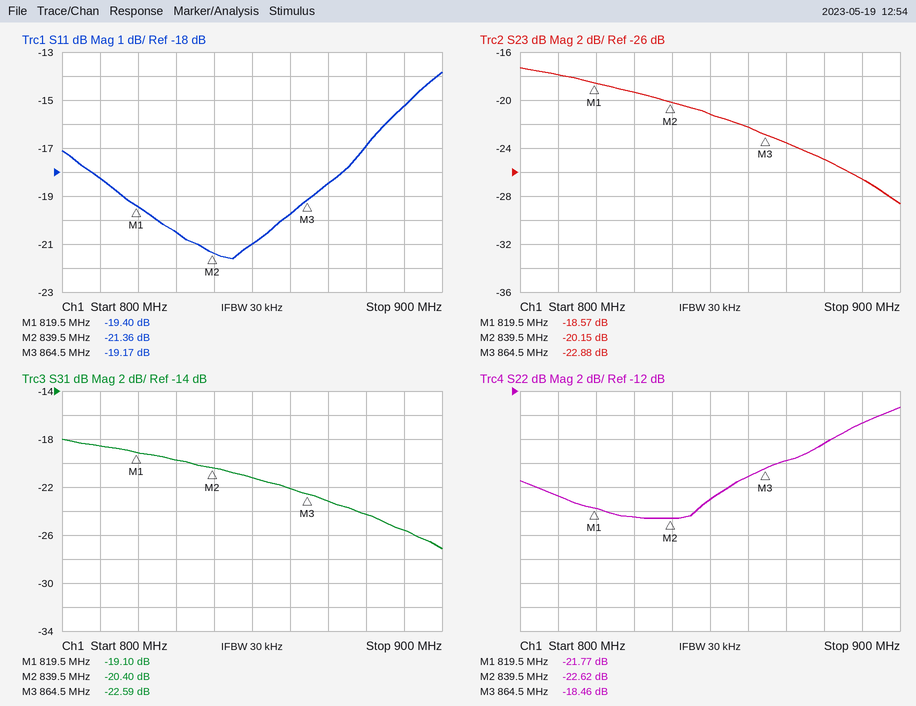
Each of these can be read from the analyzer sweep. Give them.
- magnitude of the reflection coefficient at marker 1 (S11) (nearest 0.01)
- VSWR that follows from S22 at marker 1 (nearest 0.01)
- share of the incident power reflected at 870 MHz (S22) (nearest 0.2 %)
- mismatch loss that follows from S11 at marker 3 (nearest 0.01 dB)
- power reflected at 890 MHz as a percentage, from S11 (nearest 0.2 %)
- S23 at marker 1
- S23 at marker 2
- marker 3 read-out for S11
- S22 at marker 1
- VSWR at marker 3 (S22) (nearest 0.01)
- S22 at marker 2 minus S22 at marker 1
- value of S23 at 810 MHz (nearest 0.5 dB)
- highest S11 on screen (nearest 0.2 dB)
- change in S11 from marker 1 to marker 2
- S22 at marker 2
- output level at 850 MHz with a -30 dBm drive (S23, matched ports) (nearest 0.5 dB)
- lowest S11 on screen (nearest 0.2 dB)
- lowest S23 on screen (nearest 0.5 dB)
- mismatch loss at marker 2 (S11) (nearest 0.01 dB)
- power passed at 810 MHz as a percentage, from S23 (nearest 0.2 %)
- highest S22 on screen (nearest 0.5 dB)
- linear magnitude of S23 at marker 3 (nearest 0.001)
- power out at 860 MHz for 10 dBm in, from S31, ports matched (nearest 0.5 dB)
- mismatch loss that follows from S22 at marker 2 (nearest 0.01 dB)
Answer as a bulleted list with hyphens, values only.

- 0.11
- 1.18
- 1.6 %
- 0.05 dB
- 3.0 %
- -18.57 dB
- -20.15 dB
- -19.17 dB
- -21.77 dB
- 1.27
- -0.85 dB
- -18.0 dB
- -13.8 dB
- -1.96 dB
- -22.62 dB
- -51.0 dBm
- -21.6 dB
- -28.5 dB
- 0.03 dB
- 1.6 %
- -13.5 dB
- 0.072
- -12.0 dBm
- 0.02 dB
